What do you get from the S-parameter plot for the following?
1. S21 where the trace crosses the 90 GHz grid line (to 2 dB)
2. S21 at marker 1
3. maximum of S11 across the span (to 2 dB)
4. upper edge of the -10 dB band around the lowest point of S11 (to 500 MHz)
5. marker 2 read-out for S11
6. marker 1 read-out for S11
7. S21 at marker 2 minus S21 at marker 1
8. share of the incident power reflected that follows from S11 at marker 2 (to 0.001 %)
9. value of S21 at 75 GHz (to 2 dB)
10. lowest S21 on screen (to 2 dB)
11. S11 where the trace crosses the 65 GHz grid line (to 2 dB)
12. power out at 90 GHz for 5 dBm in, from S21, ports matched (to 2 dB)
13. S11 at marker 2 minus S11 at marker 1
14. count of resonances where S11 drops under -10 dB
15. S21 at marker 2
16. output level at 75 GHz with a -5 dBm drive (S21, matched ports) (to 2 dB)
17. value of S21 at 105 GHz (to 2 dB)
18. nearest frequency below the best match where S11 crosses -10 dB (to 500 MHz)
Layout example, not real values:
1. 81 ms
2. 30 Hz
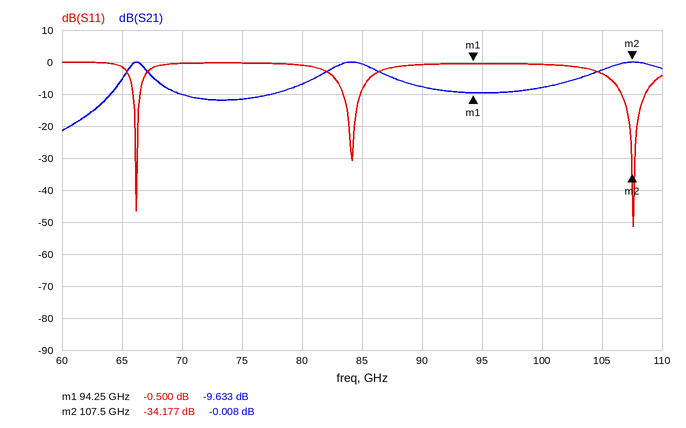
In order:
1. -8 dB
2. -9.633 dB
3. 0 dB
4. 108.5 GHz
5. -34.177 dB
6. -0.500 dB
7. 9.625 dB
8. 0.038 %
9. -12 dB
10. -22 dB
11. -2 dB
12. -2 dBm
13. -33.677 dB
14. 3
15. -0.008 dB
16. -16 dBm
17. -2 dB
18. 106.5 GHz
